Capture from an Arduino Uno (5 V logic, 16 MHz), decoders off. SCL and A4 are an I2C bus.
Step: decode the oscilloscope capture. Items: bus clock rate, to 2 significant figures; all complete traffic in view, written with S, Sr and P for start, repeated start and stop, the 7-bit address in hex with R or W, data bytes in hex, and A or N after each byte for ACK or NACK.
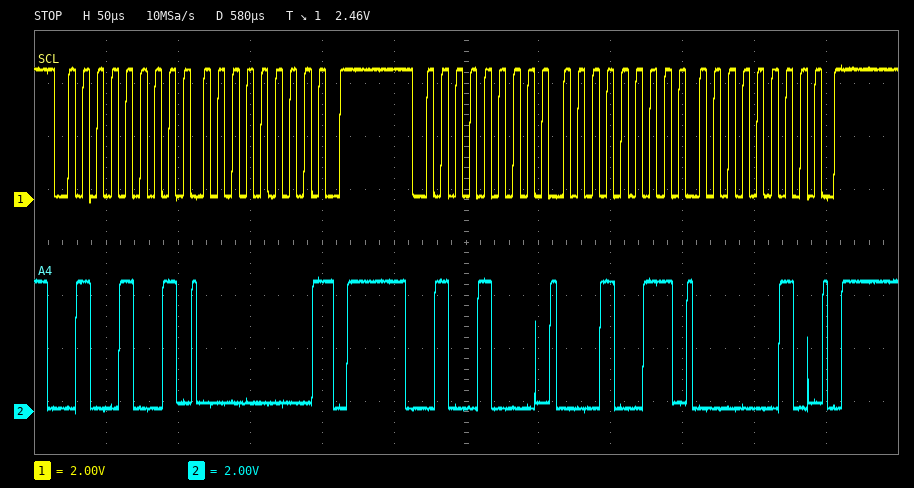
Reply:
100 kHz
S 24R A 00 N P S 24W A 13 A 02 A P
